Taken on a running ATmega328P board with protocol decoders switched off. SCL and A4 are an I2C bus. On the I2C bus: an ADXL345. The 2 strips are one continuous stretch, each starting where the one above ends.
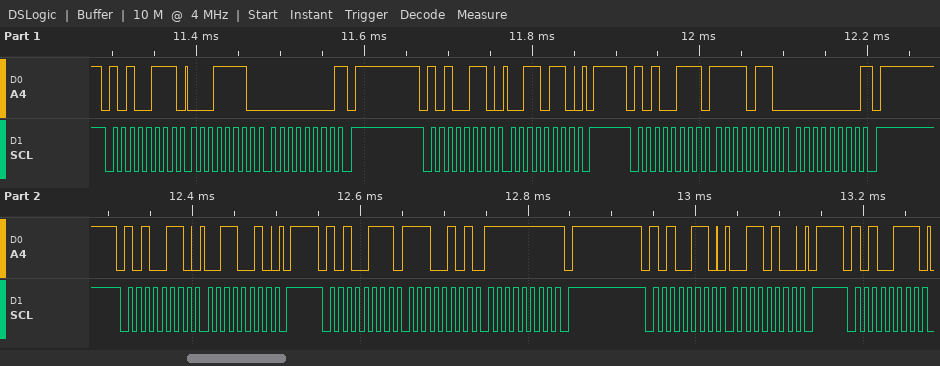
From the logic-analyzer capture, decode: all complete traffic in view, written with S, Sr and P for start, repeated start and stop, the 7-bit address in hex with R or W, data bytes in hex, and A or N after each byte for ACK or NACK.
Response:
S 53R A 1E A 00 N P S 53W A 36 A P S 53R A F6 A 00 N P S 53W A 32 A P S 53R A E5 A FF N P S 53W A 34 A P S 53R A
